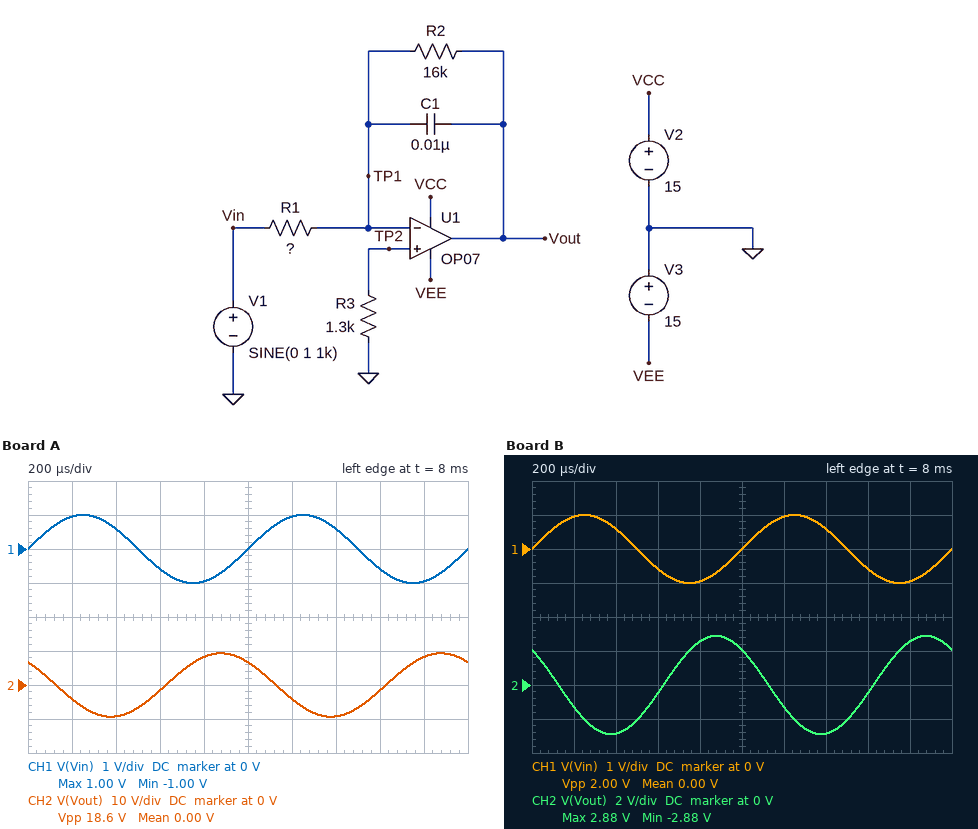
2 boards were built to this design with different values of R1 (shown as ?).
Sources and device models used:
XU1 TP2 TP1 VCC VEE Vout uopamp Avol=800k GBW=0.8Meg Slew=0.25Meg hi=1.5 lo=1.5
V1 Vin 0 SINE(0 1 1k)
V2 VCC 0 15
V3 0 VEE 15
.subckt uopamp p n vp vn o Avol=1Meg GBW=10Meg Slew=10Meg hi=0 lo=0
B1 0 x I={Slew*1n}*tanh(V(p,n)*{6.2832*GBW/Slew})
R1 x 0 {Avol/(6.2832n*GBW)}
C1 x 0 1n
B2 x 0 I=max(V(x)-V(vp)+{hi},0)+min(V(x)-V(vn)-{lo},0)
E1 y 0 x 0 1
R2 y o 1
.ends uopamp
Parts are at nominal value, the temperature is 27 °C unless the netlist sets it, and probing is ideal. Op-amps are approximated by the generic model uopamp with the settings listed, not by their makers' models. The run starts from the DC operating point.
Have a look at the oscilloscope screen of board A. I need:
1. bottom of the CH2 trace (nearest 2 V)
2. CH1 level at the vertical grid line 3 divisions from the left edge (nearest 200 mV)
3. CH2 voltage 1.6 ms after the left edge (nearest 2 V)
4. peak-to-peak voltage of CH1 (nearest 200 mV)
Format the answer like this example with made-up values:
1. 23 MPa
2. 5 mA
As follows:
1. -10 V
2. -600 mV
3. -2 V
4. 2.0 V
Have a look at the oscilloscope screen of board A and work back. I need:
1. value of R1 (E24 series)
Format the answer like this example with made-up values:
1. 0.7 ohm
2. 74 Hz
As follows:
1. 1.2 kΩ
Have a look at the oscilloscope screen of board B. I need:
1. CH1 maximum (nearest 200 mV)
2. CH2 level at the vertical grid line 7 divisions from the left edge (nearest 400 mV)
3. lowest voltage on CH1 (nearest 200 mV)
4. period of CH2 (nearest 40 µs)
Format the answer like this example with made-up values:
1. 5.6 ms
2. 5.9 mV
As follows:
1. 1.0 V
2. -2.8 V
3. -1.0 V
4. 1.00 ms
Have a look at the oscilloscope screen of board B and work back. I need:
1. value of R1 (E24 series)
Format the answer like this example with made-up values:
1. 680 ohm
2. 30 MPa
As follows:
1. 3.9 kΩ
